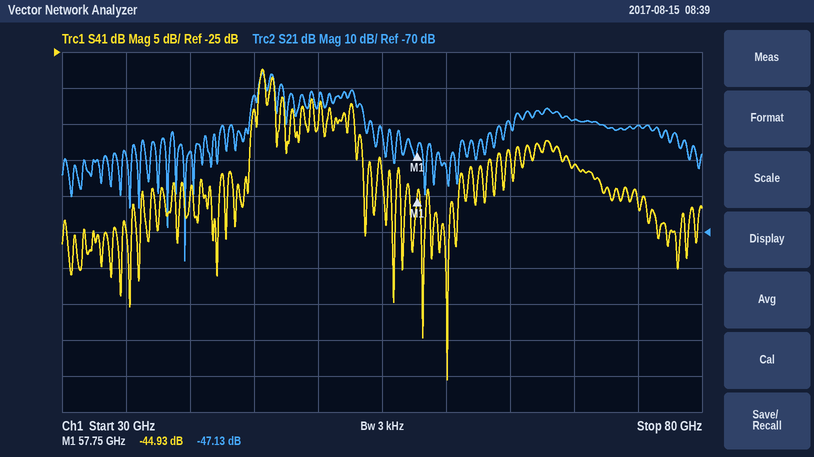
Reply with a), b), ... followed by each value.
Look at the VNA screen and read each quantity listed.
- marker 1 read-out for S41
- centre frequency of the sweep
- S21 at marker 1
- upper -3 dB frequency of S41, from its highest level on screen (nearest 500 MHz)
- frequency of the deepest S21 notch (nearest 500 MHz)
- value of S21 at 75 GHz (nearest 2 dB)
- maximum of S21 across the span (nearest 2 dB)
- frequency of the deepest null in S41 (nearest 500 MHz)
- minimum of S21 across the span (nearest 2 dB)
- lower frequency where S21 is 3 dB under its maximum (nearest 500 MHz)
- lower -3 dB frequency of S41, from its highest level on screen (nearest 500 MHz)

a) -44.93 dB
b) 55 GHz
c) -47.13 dB
d) 46.0 GHz
e) 39.5 GHz
f) -40 dB
g) -26 dB
h) 60.0 GHz
i) -78 dB
j) 45.5 GHz
k) 45.5 GHz
